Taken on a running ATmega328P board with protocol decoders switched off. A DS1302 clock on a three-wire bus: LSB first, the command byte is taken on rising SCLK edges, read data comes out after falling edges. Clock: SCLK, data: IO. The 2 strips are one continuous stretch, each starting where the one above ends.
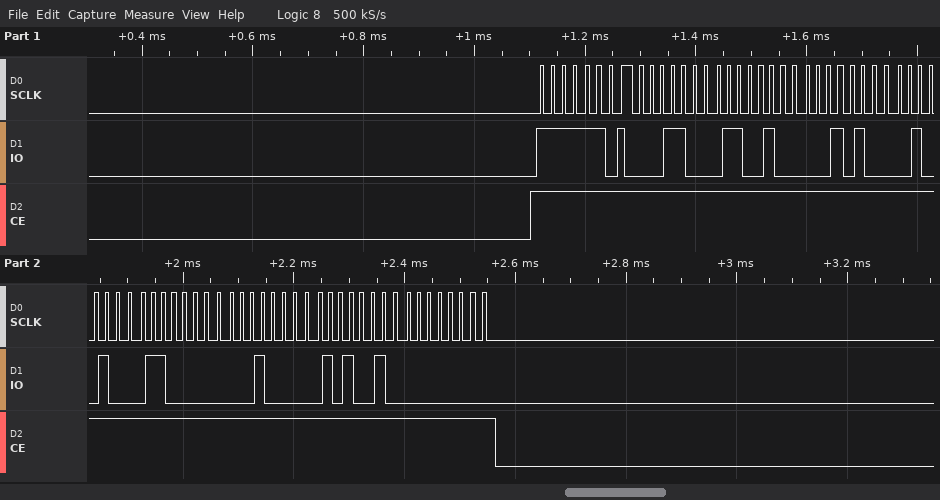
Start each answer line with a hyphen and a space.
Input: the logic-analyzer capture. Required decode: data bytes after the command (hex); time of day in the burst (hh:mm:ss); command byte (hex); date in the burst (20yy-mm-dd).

- 18 13 14 12 03 04 25 00
- 14:13:18
- 0xBF
- 2025-03-12
